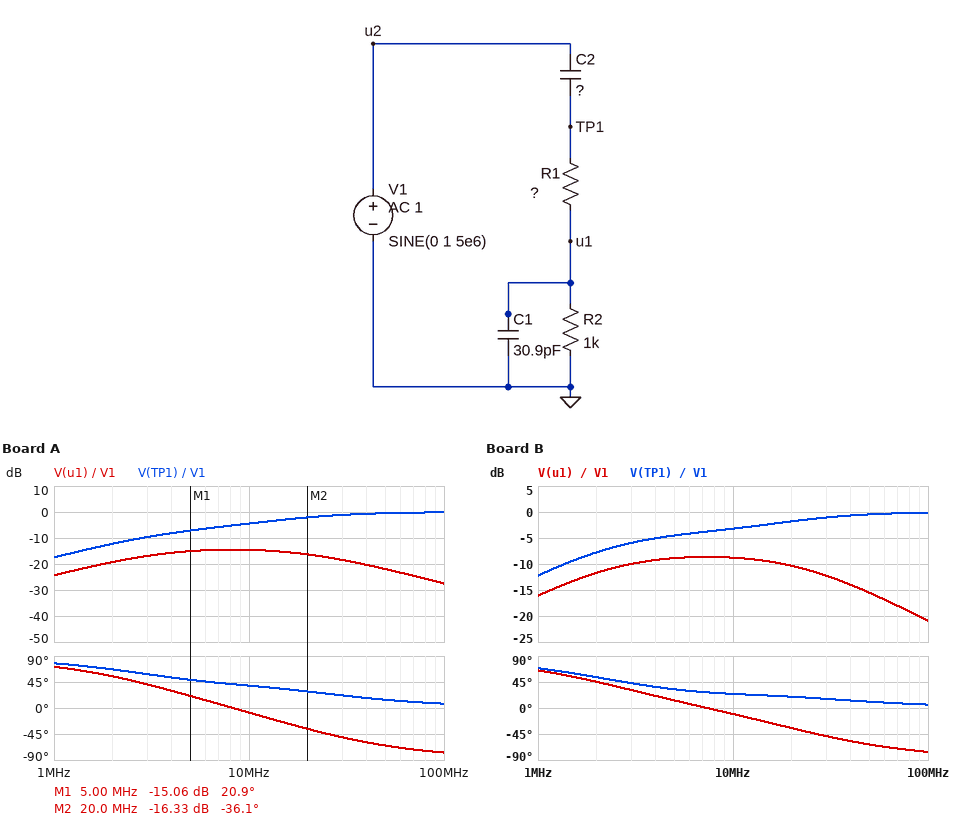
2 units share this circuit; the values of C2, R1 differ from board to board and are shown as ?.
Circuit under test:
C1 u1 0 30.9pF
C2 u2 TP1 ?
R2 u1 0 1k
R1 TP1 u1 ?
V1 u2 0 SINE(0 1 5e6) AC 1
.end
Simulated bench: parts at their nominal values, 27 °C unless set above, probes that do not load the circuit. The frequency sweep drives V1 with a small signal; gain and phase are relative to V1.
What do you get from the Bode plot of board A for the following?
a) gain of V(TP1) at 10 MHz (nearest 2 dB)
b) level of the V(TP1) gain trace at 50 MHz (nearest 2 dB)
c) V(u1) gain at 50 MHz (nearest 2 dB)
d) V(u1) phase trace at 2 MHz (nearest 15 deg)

-4 dB
0 dB
-22 dB
60 deg
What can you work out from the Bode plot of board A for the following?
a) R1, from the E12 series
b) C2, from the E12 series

1.2 kΩ
10 pF
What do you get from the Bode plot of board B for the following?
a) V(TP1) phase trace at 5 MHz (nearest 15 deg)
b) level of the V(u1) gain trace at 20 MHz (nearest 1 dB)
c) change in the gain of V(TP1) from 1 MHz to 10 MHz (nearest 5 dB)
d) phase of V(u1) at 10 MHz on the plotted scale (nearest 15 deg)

30 deg
-10 dB
10 dB
-15 deg
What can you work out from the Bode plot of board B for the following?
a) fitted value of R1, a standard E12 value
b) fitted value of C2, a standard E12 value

560 Ω
27 pF
